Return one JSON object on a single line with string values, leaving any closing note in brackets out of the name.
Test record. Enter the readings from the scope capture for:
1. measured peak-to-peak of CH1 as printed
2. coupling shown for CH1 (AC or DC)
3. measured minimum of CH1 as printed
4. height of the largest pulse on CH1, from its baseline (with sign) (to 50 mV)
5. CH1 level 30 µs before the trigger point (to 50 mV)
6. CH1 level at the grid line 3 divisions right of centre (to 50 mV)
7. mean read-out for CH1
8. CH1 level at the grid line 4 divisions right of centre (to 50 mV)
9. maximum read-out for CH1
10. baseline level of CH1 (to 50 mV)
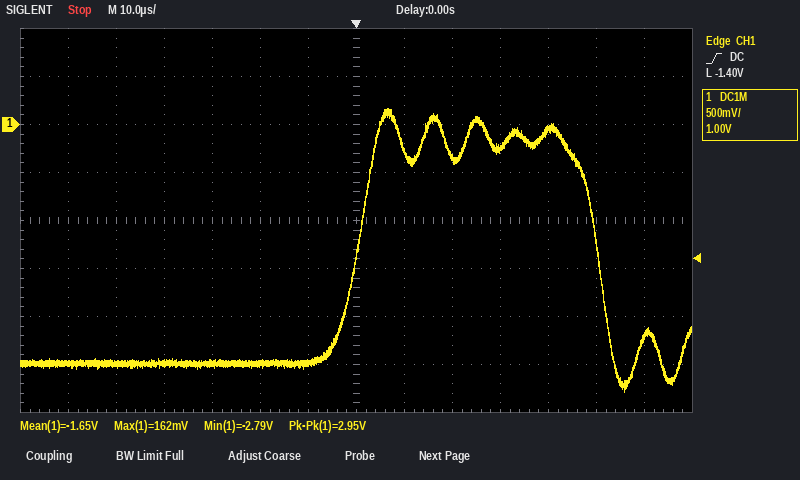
{"measured peak-to-peak of CH1 as printed": "2.95 V", "coupling shown for CH1": "DC", "measured minimum of CH1 as printed": "-2.79 V", "height of the largest pulse on CH1, from its baseline (with sign)": "+2.65 V", "CH1 level 30 µs before the trigger point": "-2.50 V", "CH1 level at the grid line 3 divisions right of centre": "-250 mV", "mean read-out for CH1": "-1.65 V", "CH1 level at the grid line 4 divisions right of centre": "-50 mV", "maximum read-out for CH1": "162 mV", "baseline level of CH1": "-2.50 V"}
